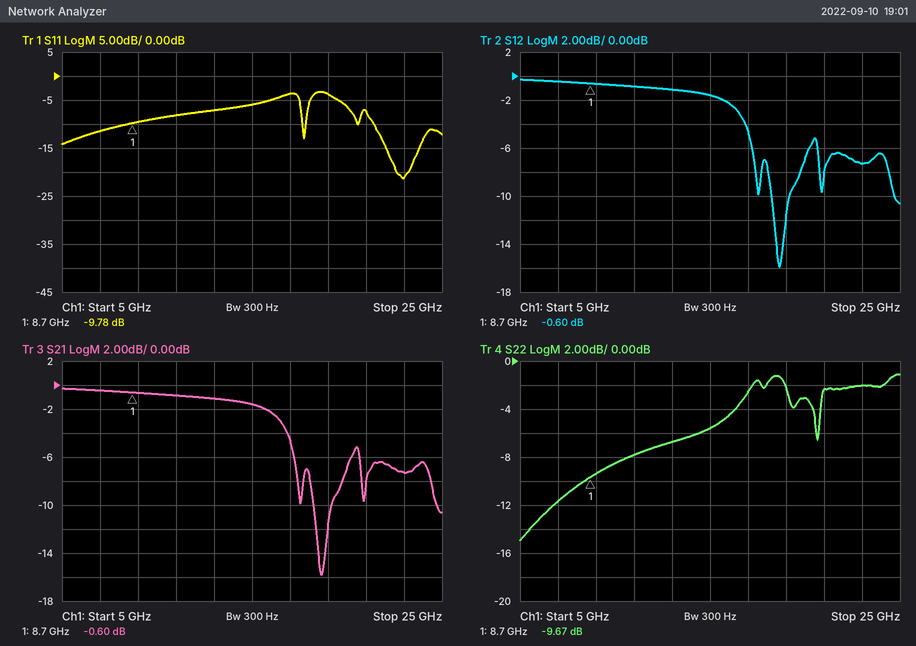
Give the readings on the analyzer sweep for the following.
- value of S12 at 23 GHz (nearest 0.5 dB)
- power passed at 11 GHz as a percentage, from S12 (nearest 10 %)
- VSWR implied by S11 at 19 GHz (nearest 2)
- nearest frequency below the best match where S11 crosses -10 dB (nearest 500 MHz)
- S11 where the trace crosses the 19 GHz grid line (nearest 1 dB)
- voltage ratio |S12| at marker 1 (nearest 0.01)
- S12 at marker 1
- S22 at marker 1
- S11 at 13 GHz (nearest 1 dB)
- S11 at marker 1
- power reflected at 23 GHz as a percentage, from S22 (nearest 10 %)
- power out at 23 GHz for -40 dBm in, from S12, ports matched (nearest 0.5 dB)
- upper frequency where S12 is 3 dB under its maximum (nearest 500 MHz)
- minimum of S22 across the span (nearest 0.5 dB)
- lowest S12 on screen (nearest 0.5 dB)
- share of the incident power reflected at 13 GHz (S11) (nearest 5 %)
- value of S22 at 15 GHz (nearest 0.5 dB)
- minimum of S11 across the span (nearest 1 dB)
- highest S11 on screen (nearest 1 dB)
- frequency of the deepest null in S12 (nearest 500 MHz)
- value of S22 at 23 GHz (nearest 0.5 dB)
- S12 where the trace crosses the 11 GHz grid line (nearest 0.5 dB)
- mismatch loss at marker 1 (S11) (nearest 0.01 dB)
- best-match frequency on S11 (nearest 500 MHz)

-7.5 dB
80 %
4
21.5 GHz
-4 dB
0.93
-0.60 dB
-9.67 dB
-7 dB
-9.78 dB
60 %
-47.5 dBm
16.5 GHz
-15.0 dB
-16.0 dB
20 %
-5.5 dB
-21 dB
-3 dB
18.5 GHz
-2.0 dB
-1.0 dB
0.48 dB
23.0 GHz
